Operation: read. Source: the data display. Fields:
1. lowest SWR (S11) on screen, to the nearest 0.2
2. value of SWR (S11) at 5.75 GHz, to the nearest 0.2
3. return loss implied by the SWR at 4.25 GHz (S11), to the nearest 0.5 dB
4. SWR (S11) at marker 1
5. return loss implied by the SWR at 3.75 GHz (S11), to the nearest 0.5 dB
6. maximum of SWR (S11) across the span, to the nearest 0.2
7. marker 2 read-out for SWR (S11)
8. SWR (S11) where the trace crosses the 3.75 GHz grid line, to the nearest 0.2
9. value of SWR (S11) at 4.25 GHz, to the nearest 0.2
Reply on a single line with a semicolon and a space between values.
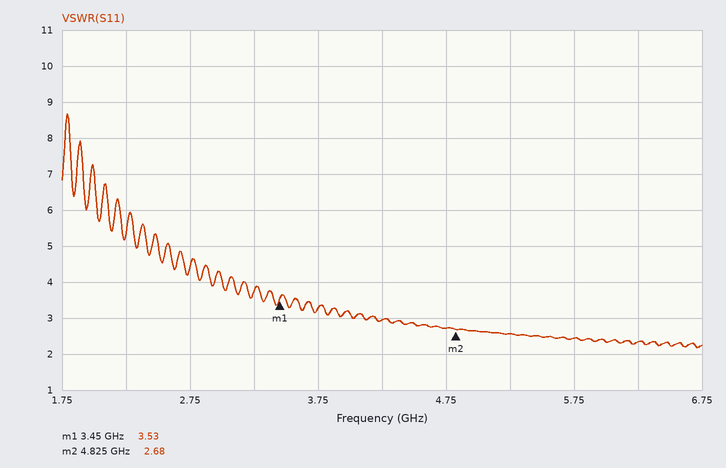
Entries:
2.2; 2.4; 6.0 dB; 3.53; 5.5 dB; 8.6; 2.68; 3.2; 3.0
